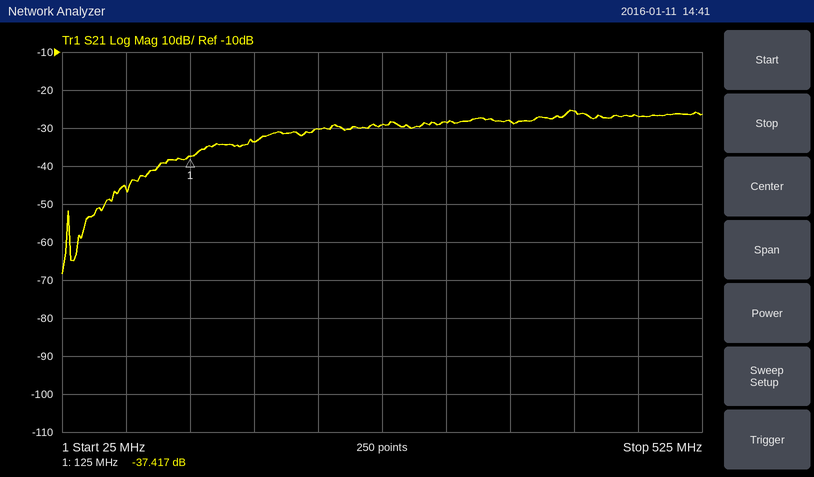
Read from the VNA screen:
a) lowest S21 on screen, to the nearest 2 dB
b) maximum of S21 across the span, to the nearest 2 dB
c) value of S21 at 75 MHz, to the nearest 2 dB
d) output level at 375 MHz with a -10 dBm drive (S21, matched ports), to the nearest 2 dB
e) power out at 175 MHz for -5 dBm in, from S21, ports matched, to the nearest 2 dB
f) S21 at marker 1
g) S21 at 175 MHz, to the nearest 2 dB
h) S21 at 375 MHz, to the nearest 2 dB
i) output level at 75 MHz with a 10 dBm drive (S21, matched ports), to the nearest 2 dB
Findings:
-68 dB
-26 dB
-46 dB
-38 dBm
-38 dBm
-37.417 dB
-34 dB
-28 dB
-36 dBm
